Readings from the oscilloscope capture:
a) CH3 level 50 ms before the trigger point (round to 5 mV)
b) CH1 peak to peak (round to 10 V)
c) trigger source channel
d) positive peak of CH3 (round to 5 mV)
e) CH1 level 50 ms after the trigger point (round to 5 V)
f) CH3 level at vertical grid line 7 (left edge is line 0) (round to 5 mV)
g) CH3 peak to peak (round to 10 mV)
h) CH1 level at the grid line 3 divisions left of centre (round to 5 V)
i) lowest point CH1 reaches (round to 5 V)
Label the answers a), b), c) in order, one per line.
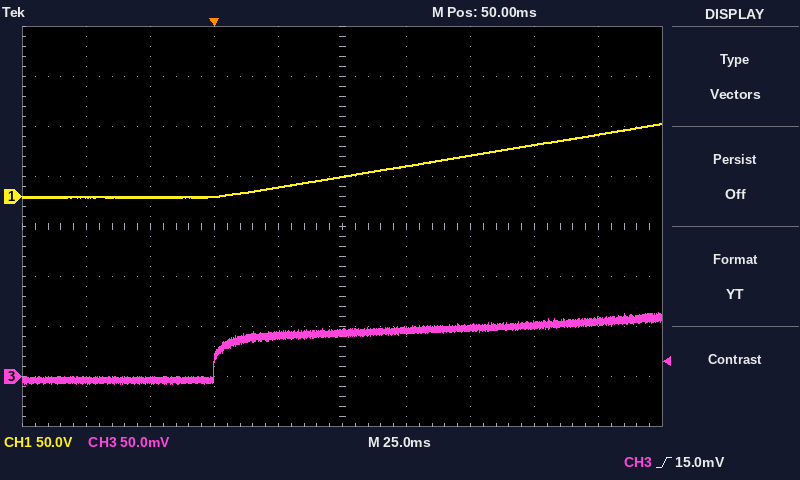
a) -5 mV
b) 70 V
c) CH3
d) 65 mV
e) 20 V
f) 50 mV
g) 70 mV
h) 0 V
i) 0 V
